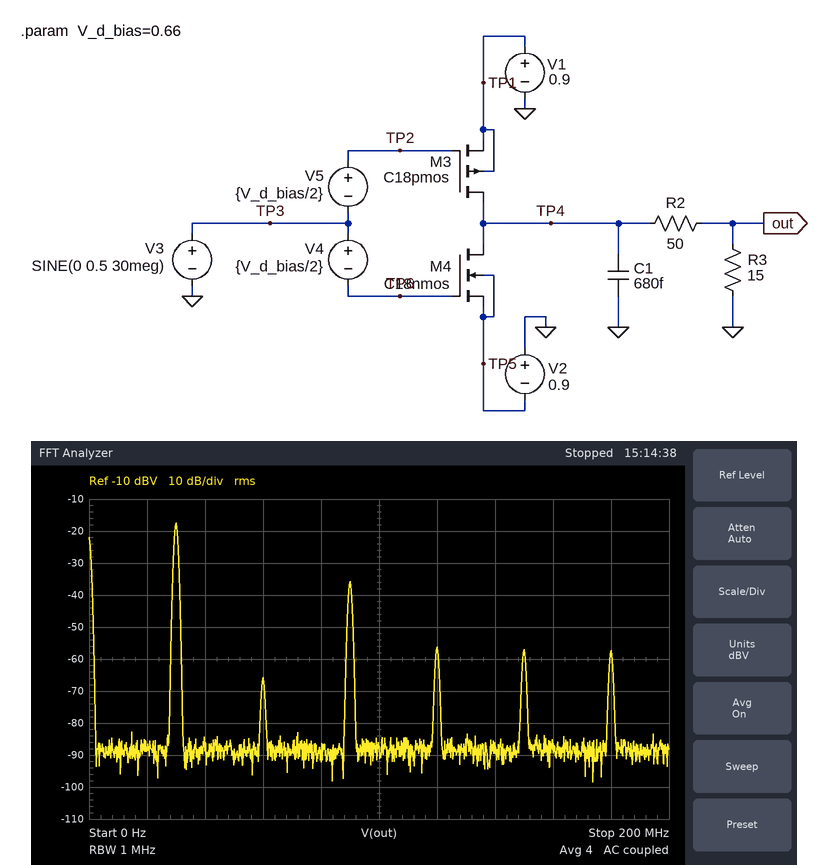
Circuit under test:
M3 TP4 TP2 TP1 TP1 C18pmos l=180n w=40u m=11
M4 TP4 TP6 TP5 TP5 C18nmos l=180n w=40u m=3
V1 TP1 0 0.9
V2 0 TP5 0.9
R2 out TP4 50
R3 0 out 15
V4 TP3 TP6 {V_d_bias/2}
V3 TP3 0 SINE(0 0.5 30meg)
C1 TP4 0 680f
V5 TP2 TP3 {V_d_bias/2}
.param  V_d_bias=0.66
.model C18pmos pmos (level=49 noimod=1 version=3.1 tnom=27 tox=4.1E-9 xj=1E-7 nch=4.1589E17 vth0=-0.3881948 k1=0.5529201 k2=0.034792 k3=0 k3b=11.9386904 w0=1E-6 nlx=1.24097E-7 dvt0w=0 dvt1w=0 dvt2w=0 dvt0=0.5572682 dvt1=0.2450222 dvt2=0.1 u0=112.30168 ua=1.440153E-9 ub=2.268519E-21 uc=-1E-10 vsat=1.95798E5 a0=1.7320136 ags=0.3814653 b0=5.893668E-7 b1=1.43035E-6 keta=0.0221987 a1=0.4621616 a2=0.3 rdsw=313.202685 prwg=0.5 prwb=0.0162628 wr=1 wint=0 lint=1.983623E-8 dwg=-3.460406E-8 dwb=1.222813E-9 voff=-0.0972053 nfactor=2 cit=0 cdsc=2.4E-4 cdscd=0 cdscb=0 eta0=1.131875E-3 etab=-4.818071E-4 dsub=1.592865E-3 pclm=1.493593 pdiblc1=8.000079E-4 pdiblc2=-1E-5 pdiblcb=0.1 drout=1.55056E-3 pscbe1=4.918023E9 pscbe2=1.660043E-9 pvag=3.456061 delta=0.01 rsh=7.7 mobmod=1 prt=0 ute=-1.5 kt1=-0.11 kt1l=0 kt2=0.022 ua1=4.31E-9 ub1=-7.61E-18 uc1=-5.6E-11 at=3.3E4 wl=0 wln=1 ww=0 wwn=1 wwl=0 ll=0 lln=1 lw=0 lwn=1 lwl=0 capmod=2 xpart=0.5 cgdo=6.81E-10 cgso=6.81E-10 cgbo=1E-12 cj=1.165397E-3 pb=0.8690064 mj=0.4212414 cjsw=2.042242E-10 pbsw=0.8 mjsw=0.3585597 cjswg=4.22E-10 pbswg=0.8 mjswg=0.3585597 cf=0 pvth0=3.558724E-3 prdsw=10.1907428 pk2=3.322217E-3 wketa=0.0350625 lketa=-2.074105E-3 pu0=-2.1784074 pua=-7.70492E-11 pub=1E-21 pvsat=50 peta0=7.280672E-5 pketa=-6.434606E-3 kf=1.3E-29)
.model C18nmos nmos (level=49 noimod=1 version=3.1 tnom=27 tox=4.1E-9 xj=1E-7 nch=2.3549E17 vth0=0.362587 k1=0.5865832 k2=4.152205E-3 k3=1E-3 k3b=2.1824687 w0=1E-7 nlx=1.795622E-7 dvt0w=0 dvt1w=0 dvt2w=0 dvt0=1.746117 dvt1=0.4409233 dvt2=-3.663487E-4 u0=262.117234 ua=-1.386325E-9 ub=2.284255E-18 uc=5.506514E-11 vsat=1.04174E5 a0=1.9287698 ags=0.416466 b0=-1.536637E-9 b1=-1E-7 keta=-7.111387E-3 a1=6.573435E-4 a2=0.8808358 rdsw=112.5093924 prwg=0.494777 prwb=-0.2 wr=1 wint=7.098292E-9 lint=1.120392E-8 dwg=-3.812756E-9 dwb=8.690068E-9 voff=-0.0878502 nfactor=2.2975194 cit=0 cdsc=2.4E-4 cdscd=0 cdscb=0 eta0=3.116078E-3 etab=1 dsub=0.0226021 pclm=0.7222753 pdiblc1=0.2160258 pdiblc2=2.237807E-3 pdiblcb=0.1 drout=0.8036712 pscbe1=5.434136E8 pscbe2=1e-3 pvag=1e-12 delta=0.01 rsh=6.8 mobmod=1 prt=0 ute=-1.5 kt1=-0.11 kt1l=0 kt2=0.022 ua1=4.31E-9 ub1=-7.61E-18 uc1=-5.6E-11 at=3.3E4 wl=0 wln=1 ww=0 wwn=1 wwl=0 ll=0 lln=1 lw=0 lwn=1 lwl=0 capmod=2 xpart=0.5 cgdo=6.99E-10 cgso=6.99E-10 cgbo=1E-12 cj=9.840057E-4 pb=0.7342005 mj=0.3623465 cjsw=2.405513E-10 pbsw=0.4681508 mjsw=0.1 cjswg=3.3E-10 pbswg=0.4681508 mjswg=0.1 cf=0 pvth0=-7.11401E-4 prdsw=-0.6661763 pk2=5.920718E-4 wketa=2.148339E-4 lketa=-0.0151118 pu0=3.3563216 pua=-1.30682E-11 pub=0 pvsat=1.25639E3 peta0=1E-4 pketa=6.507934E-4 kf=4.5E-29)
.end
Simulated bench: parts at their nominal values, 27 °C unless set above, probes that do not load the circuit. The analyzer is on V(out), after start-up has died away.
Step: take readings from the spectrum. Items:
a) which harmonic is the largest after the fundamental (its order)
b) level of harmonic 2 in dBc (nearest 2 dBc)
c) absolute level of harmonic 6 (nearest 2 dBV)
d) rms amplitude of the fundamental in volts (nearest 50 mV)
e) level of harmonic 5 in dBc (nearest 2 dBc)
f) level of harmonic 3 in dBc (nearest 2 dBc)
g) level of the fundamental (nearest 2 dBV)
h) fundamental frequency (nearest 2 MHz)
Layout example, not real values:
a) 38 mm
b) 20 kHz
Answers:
a) 3
b) -48 dBc
c) -58 dBV
d) 150 mV
e) -40 dBc
f) -18 dBc
g) -18 dBV
h) 30 MHz
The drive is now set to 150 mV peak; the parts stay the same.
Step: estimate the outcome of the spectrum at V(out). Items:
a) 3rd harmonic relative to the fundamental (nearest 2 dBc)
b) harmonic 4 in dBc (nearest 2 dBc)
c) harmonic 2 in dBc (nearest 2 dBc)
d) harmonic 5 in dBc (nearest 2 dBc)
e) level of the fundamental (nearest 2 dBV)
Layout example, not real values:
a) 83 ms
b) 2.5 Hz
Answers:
a) -34 dBc
b) -58 dBc
c) -30 dBc
d) -50 dBc
e) -26 dBV
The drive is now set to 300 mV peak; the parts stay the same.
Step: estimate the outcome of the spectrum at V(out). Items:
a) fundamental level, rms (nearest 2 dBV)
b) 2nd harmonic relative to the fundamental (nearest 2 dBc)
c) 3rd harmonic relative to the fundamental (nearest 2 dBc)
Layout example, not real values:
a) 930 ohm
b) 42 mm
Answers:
a) -20 dBV
b) -30 dBc
c) -42 dBc
